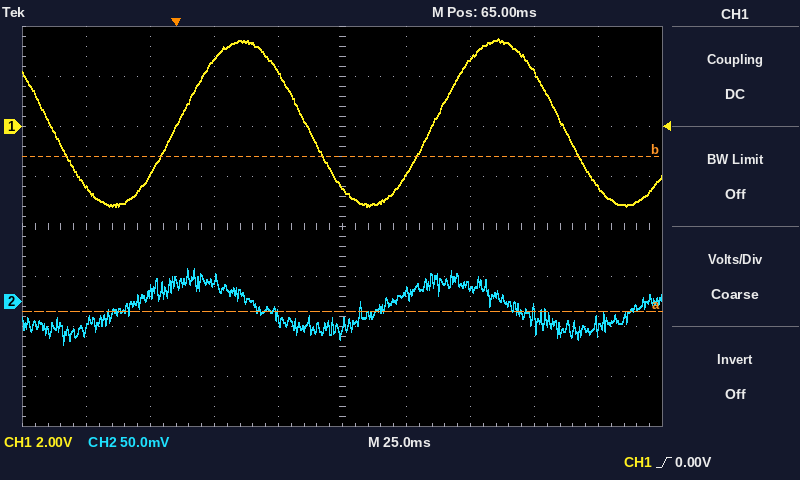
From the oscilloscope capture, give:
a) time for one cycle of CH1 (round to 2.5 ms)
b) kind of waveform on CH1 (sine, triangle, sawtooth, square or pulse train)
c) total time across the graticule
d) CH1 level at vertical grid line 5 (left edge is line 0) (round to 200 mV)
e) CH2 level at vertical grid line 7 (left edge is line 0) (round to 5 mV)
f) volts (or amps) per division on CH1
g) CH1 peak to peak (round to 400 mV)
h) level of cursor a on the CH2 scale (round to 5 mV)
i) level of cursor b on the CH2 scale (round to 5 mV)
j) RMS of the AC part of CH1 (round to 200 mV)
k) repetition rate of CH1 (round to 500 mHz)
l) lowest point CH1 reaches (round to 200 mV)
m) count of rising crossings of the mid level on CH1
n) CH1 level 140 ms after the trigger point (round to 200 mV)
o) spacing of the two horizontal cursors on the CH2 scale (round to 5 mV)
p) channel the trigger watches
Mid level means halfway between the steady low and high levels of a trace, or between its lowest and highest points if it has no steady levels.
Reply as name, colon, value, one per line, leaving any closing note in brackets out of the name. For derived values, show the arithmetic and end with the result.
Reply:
time for one cycle of CH1: 100.0 ms
kind of waveform on CH1: sine
total time across the graticule: 250 ms
CH1 level at vertical grid line 5 (left edge is line 0): -2.4 V
CH2 level at vertical grid line 7 (left edge is line 0): 15 mV
volts (or amps) per division on CH1: 2 V
CH1 peak to peak: 6.8 V
level of cursor a on the CH2 scale: -10 mV
level of cursor b on the CH2 scale: 145 mV
RMS of the AC part of CH1: 6.8 V / (2√2) ≈ 2.4 V
repetition rate of CH1: 1 / 100.0 ms ≈ 10.0 Hz
lowest point CH1 reaches: -3.2 V
count of rising crossings of the mid level on CH1: 2
CH1 level 140 ms after the trigger point: 2.2 V
spacing of the two horizontal cursors on the CH2 scale: 155 mV
channel the trigger watches: CH1
